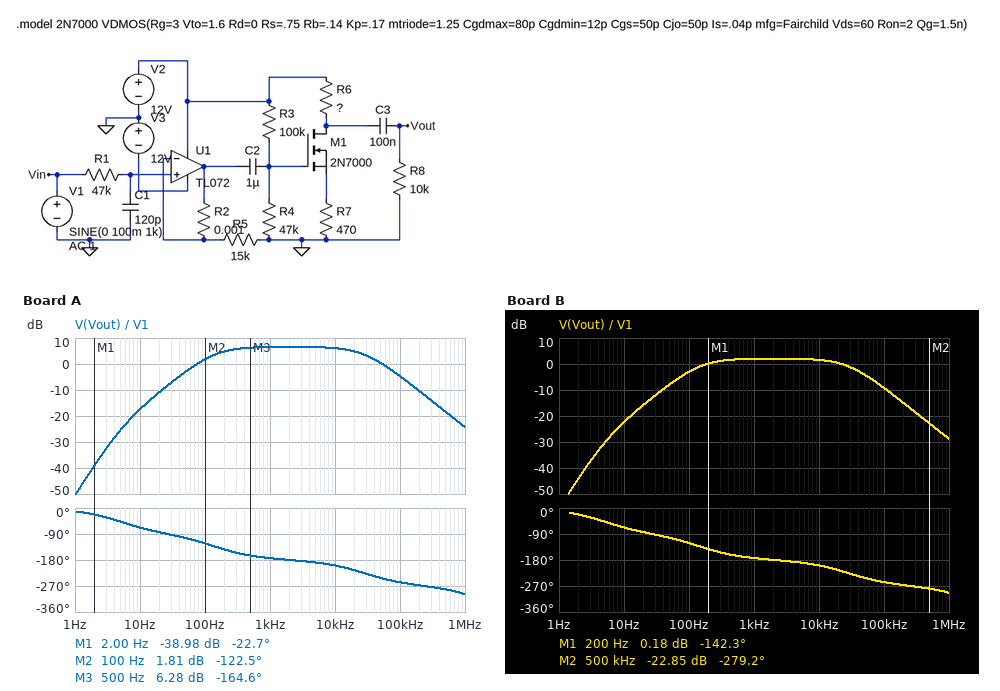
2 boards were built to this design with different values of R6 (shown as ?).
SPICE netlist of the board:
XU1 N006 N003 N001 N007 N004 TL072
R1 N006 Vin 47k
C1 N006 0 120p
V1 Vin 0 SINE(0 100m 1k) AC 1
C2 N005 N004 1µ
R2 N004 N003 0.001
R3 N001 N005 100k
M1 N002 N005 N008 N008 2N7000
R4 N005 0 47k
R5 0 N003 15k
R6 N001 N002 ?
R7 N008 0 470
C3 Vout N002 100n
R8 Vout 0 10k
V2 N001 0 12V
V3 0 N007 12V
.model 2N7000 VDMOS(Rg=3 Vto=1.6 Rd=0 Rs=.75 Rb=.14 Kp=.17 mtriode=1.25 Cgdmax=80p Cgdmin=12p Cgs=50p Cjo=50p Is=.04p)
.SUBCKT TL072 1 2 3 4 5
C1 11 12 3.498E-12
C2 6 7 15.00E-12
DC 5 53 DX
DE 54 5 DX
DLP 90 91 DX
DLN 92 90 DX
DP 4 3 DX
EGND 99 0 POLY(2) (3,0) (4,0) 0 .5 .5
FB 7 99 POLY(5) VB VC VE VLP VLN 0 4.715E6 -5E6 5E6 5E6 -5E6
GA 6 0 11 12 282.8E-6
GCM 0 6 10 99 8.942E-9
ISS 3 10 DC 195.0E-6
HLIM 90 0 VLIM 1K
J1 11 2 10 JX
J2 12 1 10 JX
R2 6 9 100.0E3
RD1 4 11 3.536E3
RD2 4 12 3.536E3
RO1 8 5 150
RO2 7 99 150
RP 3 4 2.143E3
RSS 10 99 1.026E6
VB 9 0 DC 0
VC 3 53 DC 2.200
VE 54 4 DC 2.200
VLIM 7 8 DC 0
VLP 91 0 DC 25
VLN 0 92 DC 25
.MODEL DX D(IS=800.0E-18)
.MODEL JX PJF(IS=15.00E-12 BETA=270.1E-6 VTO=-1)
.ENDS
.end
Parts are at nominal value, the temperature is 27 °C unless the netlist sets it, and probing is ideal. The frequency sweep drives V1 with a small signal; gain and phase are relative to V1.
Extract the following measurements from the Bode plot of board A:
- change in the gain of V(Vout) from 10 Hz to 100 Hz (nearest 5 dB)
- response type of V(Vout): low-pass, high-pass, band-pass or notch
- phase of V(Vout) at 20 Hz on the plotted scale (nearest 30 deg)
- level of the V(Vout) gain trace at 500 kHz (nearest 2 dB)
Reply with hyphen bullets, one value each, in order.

- 20 dB
- band-pass
- -90 deg
- -18 dB
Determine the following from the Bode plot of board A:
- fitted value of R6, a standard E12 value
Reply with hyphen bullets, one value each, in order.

- 1.2 kΩ
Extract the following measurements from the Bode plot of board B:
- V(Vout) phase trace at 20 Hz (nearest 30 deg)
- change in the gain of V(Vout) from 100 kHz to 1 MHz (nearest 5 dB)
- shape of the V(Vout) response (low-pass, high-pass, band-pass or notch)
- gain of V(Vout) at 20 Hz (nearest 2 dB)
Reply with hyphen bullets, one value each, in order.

- -90 deg
- -20 dB
- band-pass
- -16 dB
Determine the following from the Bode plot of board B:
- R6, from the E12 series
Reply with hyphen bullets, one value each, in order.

- 680 Ω
